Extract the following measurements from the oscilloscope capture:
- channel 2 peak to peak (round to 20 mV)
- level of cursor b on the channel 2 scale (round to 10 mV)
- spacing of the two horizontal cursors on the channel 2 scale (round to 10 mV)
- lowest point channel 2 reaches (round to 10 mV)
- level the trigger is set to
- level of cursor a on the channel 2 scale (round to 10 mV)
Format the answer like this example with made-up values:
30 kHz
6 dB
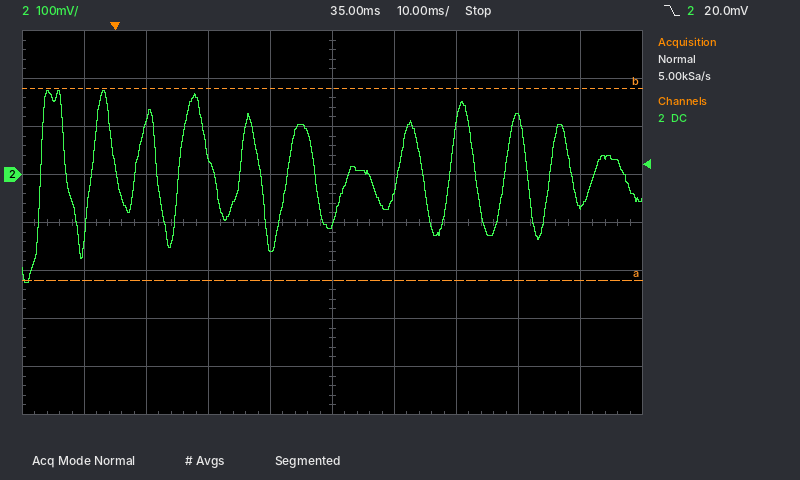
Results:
400 mV
180 mV
400 mV
-220 mV
20.0 mV
-220 mV
